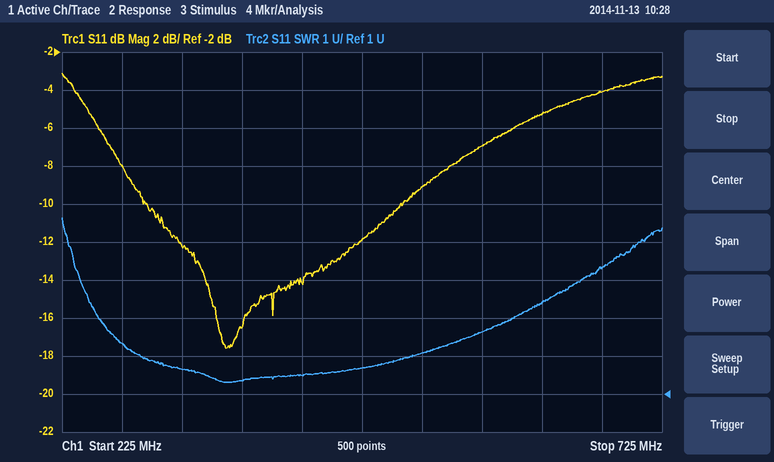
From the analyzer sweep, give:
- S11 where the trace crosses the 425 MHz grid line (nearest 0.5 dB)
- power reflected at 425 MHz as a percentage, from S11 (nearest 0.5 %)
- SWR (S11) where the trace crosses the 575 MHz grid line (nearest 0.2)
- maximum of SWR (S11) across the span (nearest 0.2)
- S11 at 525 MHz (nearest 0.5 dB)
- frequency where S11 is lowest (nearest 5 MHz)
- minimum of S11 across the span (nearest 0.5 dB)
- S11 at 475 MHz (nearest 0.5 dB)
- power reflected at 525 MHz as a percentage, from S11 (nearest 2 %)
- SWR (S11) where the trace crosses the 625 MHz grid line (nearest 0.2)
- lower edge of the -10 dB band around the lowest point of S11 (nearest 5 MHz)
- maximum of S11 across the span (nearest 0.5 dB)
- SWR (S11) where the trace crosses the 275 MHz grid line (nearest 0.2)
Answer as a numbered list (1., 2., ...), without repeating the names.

1. -14.0 dB
2. 4.0 %
3. 2.6
4. 5.6
5. -9.0 dB
6. 360 MHz
7. -17.5 dB
8. -12.0 dB
9. 12 %
10. 3.4
11. 295 MHz
12. -3.0 dB
13. 2.4
